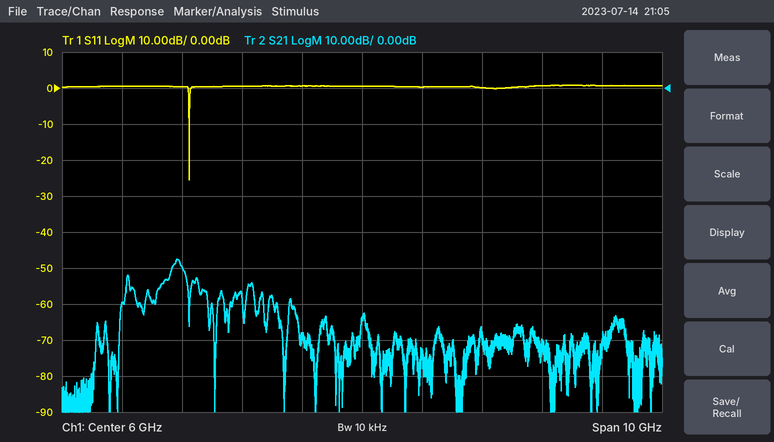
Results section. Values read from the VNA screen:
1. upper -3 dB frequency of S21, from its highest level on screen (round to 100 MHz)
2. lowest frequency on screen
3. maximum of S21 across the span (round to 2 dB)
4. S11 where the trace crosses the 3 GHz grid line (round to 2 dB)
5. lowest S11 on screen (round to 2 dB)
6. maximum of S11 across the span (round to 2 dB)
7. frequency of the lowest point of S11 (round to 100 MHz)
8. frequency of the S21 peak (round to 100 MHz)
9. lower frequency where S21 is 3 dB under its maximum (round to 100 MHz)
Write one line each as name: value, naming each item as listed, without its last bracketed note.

upper -3 dB frequency of S21, from its highest level on screen: 3.0 GHz
lowest frequency on screen: 1 GHz
maximum of S21 across the span: -48 dB
S11 where the trace crosses the 3 GHz grid line: 0 dB
lowest S11 on screen: -26 dB
maximum of S11 across the span: 0 dB
frequency of the lowest point of S11: 3.1 GHz
frequency of the S21 peak: 2.9 GHz
lower frequency where S21 is 3 dB under its maximum: 2.8 GHz
